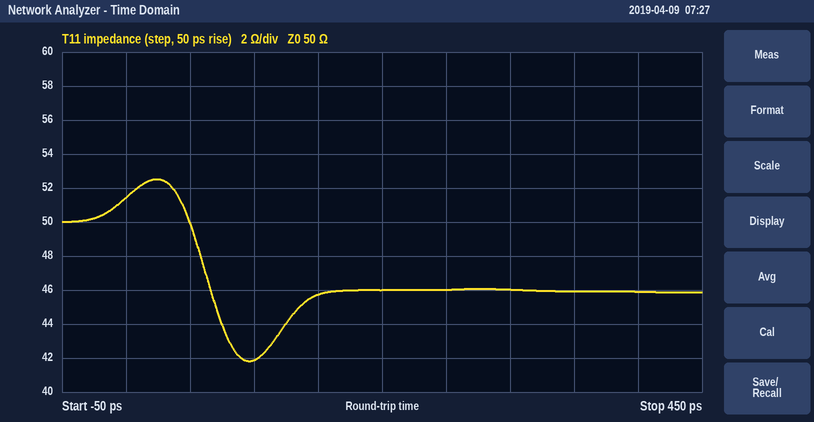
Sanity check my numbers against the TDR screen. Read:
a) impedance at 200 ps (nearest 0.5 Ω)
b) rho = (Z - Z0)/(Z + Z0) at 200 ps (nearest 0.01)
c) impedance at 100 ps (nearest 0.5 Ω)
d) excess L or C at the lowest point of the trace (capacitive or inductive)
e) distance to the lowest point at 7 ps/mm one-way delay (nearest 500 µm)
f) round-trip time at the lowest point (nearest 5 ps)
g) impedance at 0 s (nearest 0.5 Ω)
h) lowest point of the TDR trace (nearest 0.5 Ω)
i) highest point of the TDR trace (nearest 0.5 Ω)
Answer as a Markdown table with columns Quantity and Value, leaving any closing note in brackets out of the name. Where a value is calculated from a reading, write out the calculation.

| Quantity | Value |
|---|---|
| impedance at 200 ps | 46.0 Ω |
| rho = (Z - Z0)/(Z + Z0) at 200 ps | (46 − 50)/(46 + 50) ≈ -0.04 |
| impedance at 100 ps | 42.0 Ω |
| excess L or C at the lowest point of the trace | capacitive |
| distance to the lowest point at 7 ps/mm one-way delay | 95 ps / 2 / 7 ps/mm ≈ 6.79 mm, so 7.0 mm to the nearest 500 µm |
| round-trip time at the lowest point | 95 ps |
| impedance at 0 s | 51.5 Ω |
| lowest point of the TDR trace | 42.0 Ω |
| highest point of the TDR trace | 52.5 Ω |
